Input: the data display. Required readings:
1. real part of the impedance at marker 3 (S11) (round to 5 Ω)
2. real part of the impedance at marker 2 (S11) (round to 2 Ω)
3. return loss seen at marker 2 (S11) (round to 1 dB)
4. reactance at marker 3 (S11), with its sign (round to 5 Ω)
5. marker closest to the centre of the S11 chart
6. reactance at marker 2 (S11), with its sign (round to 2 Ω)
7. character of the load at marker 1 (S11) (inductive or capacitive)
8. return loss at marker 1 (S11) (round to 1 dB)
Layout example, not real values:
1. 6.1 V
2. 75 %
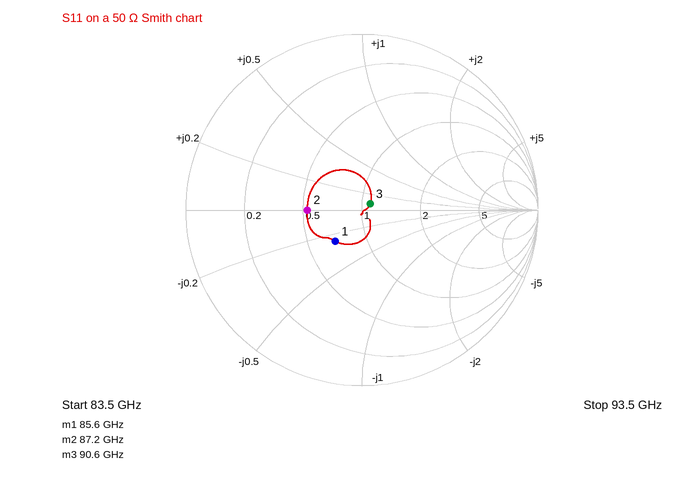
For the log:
1. 55 Ω
2. 26 Ω
3. 10 dB
4. +5 Ω
5. marker 3
6. 0 Ω
7. capacitive
8. 13 dB
